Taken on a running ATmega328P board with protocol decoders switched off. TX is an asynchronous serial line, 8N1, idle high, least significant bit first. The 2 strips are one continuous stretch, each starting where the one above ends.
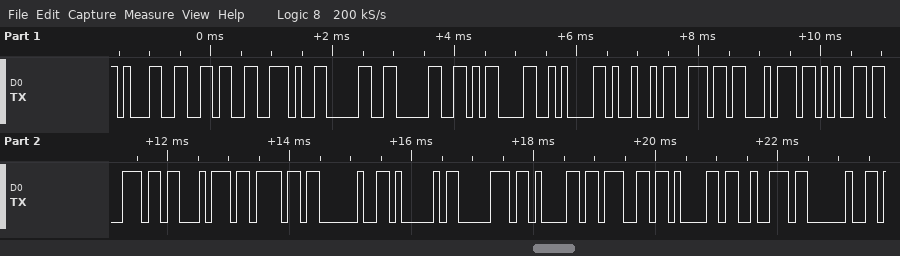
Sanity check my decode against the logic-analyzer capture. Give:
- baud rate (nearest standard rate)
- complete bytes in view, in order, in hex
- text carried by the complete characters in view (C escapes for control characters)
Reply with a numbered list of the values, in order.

1. 9600 baud
2. 31 36 2E 30 30 0D 0A 49 6E 74 65 6E 74 6F 20 41 70 61 67 61 72 20
3. "16.00\r\nIntento Apagar "
